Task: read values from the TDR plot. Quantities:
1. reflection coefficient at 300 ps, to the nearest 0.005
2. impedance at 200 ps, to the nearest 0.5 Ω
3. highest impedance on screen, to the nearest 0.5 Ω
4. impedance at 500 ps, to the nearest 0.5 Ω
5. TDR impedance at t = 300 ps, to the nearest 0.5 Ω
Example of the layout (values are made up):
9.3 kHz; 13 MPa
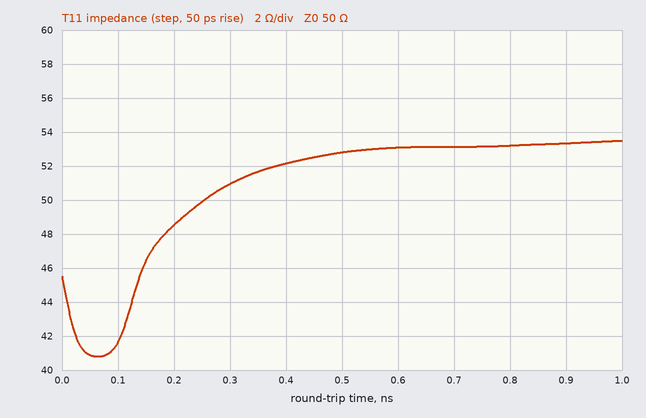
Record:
+0.010; 48.5 Ω; 53.5 Ω; 53.0 Ω; 51.0 Ω
